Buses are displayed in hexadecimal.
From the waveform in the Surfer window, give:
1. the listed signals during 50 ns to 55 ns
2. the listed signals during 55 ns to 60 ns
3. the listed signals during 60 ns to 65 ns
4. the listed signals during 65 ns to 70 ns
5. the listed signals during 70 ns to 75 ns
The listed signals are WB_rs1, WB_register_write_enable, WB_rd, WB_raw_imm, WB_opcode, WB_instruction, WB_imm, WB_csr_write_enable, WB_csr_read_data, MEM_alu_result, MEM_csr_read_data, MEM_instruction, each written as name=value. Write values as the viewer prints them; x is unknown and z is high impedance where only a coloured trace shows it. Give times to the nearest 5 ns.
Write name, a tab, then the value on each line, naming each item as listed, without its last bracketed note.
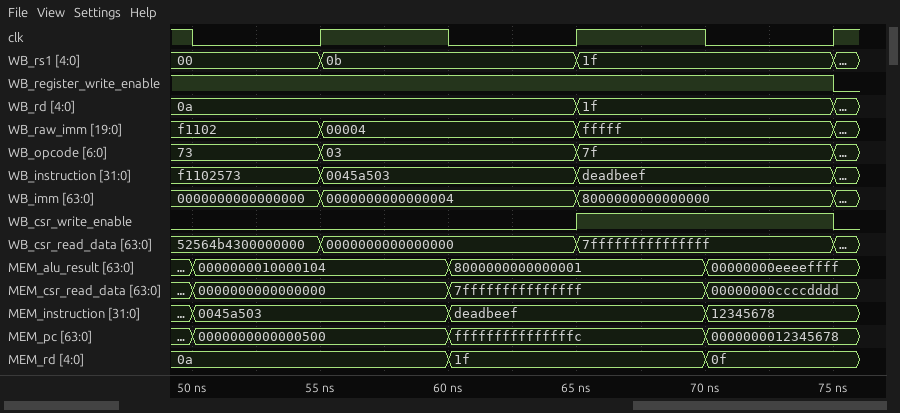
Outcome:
the listed signals during 50 ns to 55 ns	WB_rs1=00, WB_register_write_enable=1, WB_rd=0a, WB_raw_imm=f1102, WB_opcode=73, WB_instruction=f1102573, WB_imm=0000000000000000, WB_csr_write_enable=0, WB_csr_read_data=52564b4300000000, MEM_alu_result=0000000010000104, MEM_csr_read_data=0000000000000000, MEM_instruction=0045a503
the listed signals during 55 ns to 60 ns	WB_rs1=0b, WB_register_write_enable=1, WB_rd=0a, WB_raw_imm=00004, WB_opcode=03, WB_instruction=0045a503, WB_imm=0000000000000004, WB_csr_write_enable=0, WB_csr_read_data=0000000000000000, MEM_alu_result=0000000010000104, MEM_csr_read_data=0000000000000000, MEM_instruction=0045a503
the listed signals during 60 ns to 65 ns	WB_rs1=0b, WB_register_write_enable=1, WB_rd=0a, WB_raw_imm=00004, WB_opcode=03, WB_instruction=0045a503, WB_imm=0000000000000004, WB_csr_write_enable=0, WB_csr_read_data=0000000000000000, MEM_alu_result=8000000000000001, MEM_csr_read_data=7fffffffffffffff, MEM_instruction=deadbeef
the listed signals during 65 ns to 70 ns	WB_rs1=1f, WB_register_write_enable=1, WB_rd=1f, WB_raw_imm=fffff, WB_opcode=7f, WB_instruction=deadbeef, WB_imm=8000000000000000, WB_csr_write_enable=1, WB_csr_read_data=7fffffffffffffff, MEM_alu_result=8000000000000001, MEM_csr_read_data=7fffffffffffffff, MEM_instruction=deadbeef
the listed signals during 70 ns to 75 ns	WB_rs1=1f, WB_register_write_enable=1, WB_rd=1f, WB_raw_imm=fffff, WB_opcode=7f, WB_instruction=deadbeef, WB_imm=8000000000000000, WB_csr_write_enable=1, WB_csr_read_data=7fffffffffffffff, MEM_alu_result=00000000eeeeffff, MEM_csr_read_data=00000000ccccdddd, MEM_instruction=12345678
